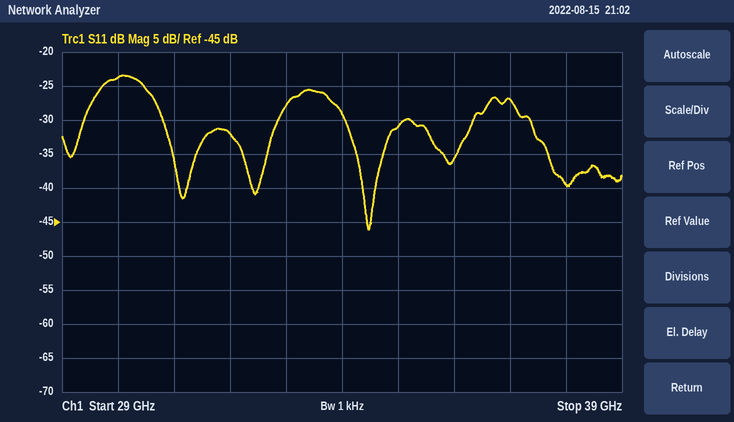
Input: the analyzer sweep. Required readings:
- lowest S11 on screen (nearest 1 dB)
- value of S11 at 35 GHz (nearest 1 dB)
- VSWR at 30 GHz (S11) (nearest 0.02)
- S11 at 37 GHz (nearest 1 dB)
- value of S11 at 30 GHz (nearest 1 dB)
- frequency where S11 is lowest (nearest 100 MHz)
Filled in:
-46 dB
-31 dB
1.14
-27 dB
-24 dB
34.5 GHz
